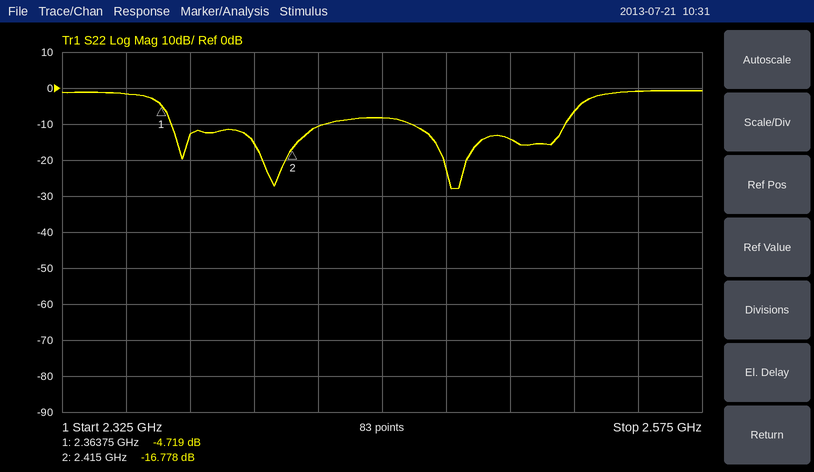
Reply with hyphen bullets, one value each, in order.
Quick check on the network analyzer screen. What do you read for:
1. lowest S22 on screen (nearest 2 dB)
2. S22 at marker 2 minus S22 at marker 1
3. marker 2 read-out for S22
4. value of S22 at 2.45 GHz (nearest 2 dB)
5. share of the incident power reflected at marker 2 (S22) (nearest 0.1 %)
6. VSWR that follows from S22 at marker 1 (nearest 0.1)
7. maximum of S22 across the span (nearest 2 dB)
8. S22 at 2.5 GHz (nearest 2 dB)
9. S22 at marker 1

- -28 dB
- -12.059 dB
- -16.778 dB
- -8 dB
- 2.1 %
- 3.8
- 0 dB
- -14 dB
- -4.719 dB
